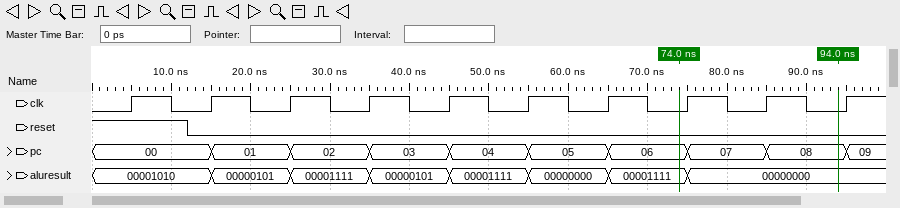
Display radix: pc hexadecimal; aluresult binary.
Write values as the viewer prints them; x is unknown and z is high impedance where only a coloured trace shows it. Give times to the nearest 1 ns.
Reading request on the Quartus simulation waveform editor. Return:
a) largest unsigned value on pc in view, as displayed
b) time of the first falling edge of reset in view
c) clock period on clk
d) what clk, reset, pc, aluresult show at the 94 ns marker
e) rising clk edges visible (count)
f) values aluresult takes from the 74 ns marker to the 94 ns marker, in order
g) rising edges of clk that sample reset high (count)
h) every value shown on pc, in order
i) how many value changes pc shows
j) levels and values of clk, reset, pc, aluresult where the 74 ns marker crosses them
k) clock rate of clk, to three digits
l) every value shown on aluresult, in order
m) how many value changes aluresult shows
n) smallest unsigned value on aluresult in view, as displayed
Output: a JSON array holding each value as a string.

["09", "12 ns", "10 ns", "clk=0, reset=0, pc=08, aluresult=00000000", "10", "00001111, 00000000", "1", "00, 01, 02, 03, 04, 05, 06, 07, 08, 09", "9", "clk=0, reset=0, pc=06, aluresult=00001111", "100 MHz", "00001010, 00000101, 00001111, 00000101, 00001111, 00000000, 00001111, 00000000", "7", "00000000"]
